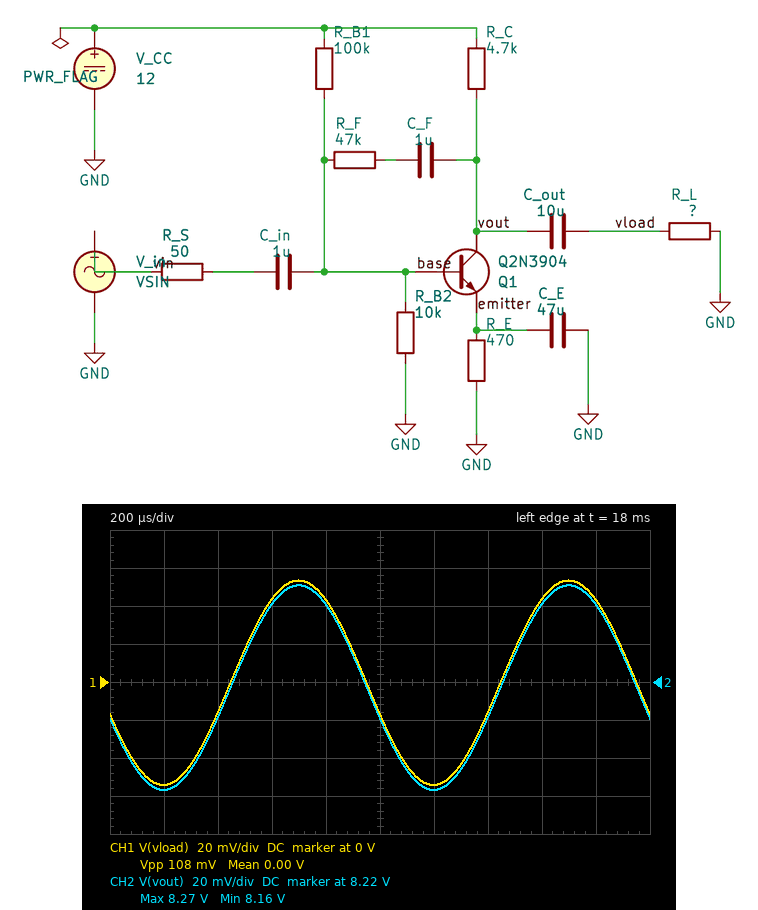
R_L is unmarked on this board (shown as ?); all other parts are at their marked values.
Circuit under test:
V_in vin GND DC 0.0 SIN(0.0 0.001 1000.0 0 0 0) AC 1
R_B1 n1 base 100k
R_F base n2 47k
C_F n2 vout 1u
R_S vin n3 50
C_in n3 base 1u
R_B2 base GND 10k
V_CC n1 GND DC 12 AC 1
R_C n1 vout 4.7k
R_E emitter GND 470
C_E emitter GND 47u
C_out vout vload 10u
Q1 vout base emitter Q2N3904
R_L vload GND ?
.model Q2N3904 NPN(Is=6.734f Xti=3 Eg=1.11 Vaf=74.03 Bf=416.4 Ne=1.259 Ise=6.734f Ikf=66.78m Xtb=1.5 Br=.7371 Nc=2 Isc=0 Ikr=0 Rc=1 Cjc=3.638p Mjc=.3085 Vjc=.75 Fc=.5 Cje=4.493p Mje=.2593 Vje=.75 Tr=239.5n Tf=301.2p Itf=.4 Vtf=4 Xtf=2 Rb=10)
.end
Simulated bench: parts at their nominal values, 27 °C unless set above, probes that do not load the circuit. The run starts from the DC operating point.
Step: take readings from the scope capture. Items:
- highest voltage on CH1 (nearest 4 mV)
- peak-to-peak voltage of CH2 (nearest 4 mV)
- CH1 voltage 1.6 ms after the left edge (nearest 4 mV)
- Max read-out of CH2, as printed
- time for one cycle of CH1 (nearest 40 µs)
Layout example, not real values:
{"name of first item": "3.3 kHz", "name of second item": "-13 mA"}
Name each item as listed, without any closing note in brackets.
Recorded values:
{"highest voltage on CH1": "52 mV", "peak-to-peak voltage of CH2": "108 mV", "CH1 voltage 1.6 ms after the left edge": "44 mV", "Max read-out of CH2, as printed": "8.27 V", "time for one cycle of CH1": "1.00 ms"}
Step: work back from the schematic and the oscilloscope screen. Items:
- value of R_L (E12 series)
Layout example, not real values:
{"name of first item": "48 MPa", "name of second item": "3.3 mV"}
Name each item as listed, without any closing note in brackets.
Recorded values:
{"value of R_L": "3.9 kΩ"}
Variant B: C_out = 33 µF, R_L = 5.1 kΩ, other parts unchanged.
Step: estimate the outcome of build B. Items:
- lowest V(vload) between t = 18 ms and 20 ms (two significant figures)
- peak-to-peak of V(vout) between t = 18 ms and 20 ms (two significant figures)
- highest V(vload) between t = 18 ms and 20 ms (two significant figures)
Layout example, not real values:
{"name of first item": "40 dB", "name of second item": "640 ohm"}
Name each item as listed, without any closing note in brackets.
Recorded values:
{"lowest V(vload) between t = 18 ms and 20 ms": "-61 mV", "peak-to-peak of V(vout) between t = 18 ms and 20 ms": "120 mV", "highest V(vload) between t = 18 ms and 20 ms": "60 mV"}
